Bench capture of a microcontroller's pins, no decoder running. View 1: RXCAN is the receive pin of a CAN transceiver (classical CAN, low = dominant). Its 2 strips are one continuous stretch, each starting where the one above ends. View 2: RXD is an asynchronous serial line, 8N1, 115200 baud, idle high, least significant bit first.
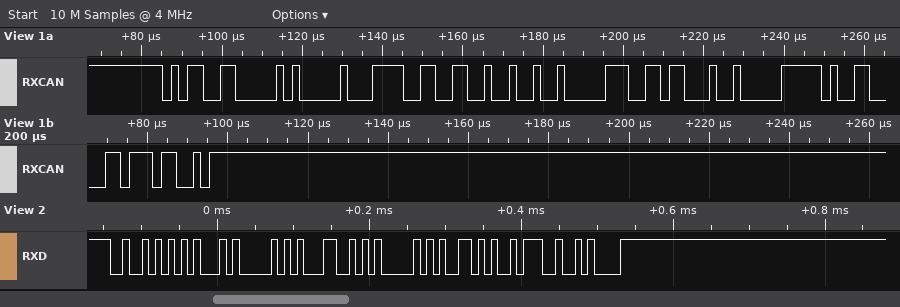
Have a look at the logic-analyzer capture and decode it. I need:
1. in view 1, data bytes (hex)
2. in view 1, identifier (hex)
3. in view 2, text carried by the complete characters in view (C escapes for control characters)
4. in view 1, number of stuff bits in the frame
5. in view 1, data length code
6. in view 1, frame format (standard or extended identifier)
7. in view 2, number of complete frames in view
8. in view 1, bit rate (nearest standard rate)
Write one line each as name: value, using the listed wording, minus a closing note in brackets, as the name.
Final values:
in view 1, data bytes: 07 99 92 48 33 62 41 F3
in view 1, identifier: 0x598
in view 2, text carried by the complete characters in view: "REPLAY:\n"
in view 1, number of stuff bits in the frame: 5
in view 1, data length code: 8
in view 1, frame format: standard
in view 2, number of complete frames in view: 8
in view 1, bit rate: 500 kbit/s
